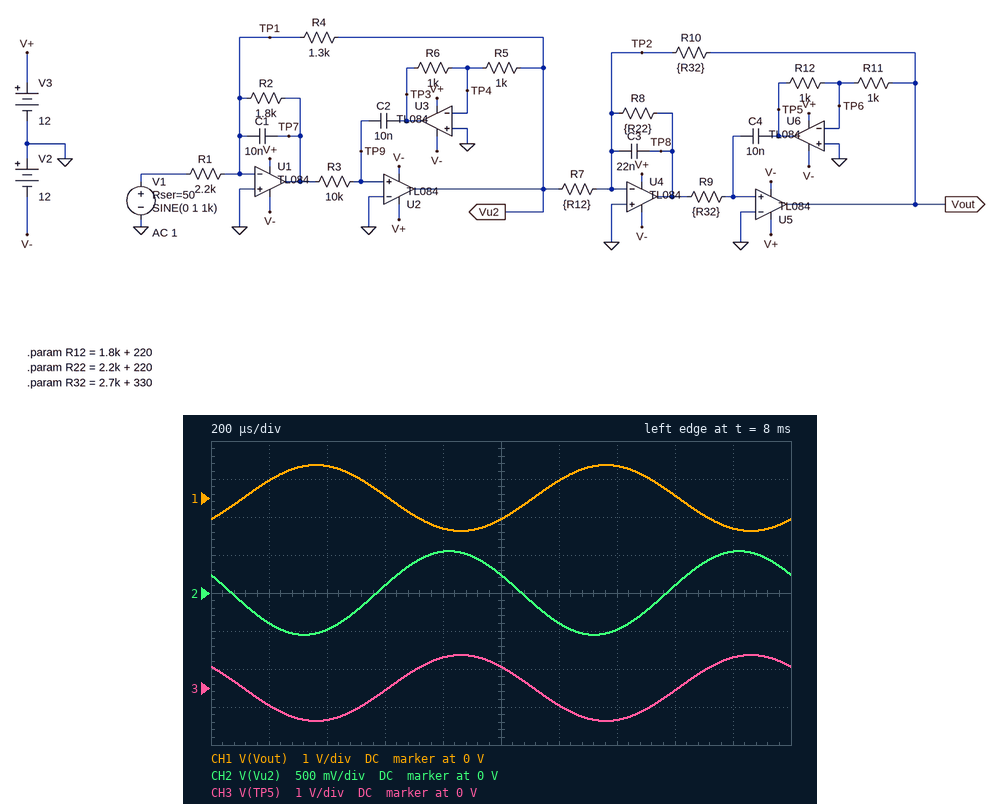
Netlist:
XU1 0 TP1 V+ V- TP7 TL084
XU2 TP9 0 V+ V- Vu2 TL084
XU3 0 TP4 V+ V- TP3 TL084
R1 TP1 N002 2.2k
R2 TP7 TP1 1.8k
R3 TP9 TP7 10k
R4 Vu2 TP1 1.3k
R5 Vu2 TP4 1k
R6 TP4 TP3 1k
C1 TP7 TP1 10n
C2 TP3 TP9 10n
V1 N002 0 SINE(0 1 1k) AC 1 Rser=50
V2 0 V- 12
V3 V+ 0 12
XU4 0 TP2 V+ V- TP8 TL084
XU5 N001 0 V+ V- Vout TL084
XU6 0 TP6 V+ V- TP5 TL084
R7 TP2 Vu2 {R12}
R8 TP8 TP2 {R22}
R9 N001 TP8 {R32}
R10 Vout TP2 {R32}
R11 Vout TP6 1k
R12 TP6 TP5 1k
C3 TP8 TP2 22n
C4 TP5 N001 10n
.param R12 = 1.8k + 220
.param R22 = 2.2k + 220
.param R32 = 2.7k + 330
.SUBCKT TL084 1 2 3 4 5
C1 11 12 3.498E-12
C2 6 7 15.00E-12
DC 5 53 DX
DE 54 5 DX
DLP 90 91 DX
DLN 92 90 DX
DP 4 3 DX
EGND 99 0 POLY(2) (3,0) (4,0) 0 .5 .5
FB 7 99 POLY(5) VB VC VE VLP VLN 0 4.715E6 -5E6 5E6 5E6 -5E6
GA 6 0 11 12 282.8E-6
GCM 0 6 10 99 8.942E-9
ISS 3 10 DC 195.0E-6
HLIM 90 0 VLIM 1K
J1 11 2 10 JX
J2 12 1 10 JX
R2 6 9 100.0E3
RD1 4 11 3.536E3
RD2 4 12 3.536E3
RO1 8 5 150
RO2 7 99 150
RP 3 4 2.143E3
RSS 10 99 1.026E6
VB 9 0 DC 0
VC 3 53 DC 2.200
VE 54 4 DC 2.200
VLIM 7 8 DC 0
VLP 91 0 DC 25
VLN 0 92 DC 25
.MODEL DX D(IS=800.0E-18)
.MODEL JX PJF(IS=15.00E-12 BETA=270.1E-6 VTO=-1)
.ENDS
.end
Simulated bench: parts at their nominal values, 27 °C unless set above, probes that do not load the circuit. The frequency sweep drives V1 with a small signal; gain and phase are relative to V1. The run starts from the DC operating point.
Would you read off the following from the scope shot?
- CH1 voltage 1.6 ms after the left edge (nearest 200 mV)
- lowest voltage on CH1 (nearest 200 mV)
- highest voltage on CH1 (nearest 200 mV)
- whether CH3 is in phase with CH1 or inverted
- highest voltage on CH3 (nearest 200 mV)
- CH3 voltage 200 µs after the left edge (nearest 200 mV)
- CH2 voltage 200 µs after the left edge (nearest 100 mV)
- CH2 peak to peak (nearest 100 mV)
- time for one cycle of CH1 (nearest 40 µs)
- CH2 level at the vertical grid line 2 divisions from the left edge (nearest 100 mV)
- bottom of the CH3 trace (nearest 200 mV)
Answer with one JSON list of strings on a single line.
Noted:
["0 V", "-800 mV", "800 mV", "inverted", "800 mV", "-400 mV", "-400 mV", "1.1 V", "1.00 ms", "-500 mV", "-800 mV"]
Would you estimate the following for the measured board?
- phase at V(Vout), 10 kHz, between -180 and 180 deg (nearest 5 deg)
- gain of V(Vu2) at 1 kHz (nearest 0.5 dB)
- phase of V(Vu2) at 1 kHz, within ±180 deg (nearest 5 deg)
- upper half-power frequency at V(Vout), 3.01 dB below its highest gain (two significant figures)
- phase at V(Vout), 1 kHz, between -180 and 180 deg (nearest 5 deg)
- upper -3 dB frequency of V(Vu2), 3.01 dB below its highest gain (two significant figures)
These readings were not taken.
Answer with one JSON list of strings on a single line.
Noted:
["65 deg", "-5.0 dB", "155 deg", "3.6 kHz", "-40 deg", "2.8 kHz"]
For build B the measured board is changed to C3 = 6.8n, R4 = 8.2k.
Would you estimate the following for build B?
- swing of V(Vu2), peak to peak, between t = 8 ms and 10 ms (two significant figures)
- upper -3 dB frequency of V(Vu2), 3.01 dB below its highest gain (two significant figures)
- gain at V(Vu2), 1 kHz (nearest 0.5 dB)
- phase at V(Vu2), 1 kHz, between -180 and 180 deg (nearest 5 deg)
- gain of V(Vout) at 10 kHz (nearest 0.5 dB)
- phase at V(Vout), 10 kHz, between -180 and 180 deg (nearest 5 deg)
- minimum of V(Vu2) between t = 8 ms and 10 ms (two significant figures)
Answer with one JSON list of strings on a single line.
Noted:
["2.5 V", "360 Hz", "2.0 dB", "105 deg", "-27.0 dB", "100 deg", "-1.2 V"]
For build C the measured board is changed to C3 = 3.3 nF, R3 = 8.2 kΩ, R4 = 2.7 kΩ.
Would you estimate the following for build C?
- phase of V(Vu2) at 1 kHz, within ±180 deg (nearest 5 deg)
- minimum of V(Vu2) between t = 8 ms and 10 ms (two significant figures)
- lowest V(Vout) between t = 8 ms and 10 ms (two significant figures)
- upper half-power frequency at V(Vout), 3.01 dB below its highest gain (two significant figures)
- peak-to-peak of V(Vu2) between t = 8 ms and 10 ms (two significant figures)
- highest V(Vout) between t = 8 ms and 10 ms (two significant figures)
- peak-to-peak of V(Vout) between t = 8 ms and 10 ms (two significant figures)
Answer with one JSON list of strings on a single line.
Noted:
["140 deg", "-1.0 V", "-1.5 V", "1.4 kHz", "2.0 V", "1.5 V", "3.0 V"]
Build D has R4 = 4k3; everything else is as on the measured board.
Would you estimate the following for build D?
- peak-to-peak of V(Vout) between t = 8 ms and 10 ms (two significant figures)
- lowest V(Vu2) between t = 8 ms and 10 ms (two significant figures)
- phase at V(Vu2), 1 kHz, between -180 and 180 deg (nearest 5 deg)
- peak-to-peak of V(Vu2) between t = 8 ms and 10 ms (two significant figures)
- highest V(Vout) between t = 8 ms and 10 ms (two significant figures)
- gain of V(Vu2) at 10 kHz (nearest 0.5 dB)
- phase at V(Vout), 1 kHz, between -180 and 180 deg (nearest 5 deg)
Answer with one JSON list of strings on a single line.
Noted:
["3.5 V", "-1.1 V", "120 deg", "2.2 V", "1.8 V", "-21.0 dB", "-75 deg"]
